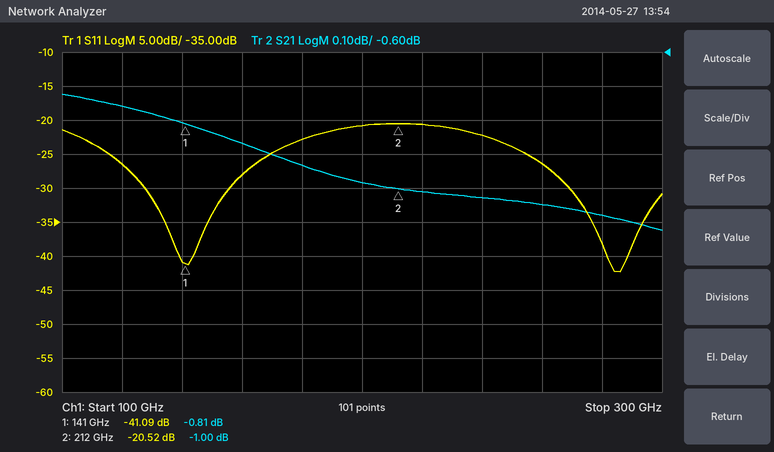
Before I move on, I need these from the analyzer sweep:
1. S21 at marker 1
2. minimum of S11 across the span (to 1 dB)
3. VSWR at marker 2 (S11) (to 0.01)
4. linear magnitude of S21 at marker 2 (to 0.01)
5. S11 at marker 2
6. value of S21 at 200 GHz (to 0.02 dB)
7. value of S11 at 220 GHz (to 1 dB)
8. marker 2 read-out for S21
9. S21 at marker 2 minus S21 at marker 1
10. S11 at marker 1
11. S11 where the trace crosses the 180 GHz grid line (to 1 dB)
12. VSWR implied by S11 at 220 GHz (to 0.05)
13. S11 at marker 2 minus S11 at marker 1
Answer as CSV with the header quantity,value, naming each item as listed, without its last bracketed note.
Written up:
quantity,value
S21 at marker 1,-0.81 dB
minimum of S11 across the span,-42 dB
VSWR at marker 2 (S11),1.21
linear magnitude of S21 at marker 2,0.89
S11 at marker 2,-20.52 dB
value of S21 at 200 GHz,-0.98 dB
value of S11 at 220 GHz,-21 dB
marker 2 read-out for S21,-1.00 dB
S21 at marker 2 minus S21 at marker 1,-0.19 dB
S11 at marker 1,-41.09 dB
S11 where the trace crosses the 180 GHz grid line,-23 dB
VSWR implied by S11 at 220 GHz,1.20
S11 at marker 2 minus S11 at marker 1,20.57 dB
